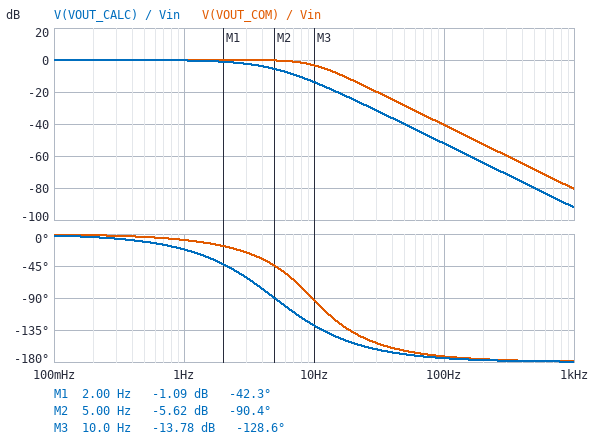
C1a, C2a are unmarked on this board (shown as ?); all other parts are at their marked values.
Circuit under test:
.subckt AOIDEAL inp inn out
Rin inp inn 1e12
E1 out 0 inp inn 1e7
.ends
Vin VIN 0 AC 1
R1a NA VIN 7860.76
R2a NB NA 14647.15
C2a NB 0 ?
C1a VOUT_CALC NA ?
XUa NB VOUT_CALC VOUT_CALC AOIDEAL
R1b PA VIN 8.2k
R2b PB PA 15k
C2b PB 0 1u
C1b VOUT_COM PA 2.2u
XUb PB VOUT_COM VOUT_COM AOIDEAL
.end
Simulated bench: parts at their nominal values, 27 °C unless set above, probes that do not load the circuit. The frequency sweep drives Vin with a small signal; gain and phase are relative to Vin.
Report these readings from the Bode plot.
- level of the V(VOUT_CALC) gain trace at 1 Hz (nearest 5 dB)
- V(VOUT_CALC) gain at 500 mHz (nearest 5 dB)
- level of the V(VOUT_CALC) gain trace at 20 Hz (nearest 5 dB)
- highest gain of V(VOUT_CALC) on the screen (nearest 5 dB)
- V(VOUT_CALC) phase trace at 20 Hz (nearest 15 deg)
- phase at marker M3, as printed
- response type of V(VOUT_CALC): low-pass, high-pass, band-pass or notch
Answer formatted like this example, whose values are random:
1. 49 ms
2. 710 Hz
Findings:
1. 0 dB
2. 0 dB
3. -25 dB
4. 0 dB
5. -150 deg
6. -128.6 deg
7. low-pass
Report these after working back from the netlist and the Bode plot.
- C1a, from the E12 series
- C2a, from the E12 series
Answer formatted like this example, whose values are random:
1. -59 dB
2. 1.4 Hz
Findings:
1. 3.3 µF
2. 2.7 µF
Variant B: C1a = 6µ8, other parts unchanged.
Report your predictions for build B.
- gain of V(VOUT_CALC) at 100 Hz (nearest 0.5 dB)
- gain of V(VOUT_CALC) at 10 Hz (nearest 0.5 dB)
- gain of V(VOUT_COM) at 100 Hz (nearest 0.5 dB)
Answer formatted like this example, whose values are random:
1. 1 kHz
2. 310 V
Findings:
1. -58.5 dB
2. -18.5 dB
3. -40.5 dB
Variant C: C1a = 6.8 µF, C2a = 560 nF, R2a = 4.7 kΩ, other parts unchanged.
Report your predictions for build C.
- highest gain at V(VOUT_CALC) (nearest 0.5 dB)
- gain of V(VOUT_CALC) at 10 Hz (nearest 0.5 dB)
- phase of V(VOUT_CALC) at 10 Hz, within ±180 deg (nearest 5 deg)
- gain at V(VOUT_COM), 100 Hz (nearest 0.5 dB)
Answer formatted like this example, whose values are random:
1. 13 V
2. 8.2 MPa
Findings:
1. 5.0 dB
2. 4.0 dB
3. -45 deg
4. -40.5 dB
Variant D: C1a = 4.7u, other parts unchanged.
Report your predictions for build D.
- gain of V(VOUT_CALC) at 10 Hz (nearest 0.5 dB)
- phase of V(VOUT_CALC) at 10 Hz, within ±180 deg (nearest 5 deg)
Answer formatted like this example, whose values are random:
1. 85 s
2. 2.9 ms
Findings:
1. -15.5 dB
2. -140 deg
